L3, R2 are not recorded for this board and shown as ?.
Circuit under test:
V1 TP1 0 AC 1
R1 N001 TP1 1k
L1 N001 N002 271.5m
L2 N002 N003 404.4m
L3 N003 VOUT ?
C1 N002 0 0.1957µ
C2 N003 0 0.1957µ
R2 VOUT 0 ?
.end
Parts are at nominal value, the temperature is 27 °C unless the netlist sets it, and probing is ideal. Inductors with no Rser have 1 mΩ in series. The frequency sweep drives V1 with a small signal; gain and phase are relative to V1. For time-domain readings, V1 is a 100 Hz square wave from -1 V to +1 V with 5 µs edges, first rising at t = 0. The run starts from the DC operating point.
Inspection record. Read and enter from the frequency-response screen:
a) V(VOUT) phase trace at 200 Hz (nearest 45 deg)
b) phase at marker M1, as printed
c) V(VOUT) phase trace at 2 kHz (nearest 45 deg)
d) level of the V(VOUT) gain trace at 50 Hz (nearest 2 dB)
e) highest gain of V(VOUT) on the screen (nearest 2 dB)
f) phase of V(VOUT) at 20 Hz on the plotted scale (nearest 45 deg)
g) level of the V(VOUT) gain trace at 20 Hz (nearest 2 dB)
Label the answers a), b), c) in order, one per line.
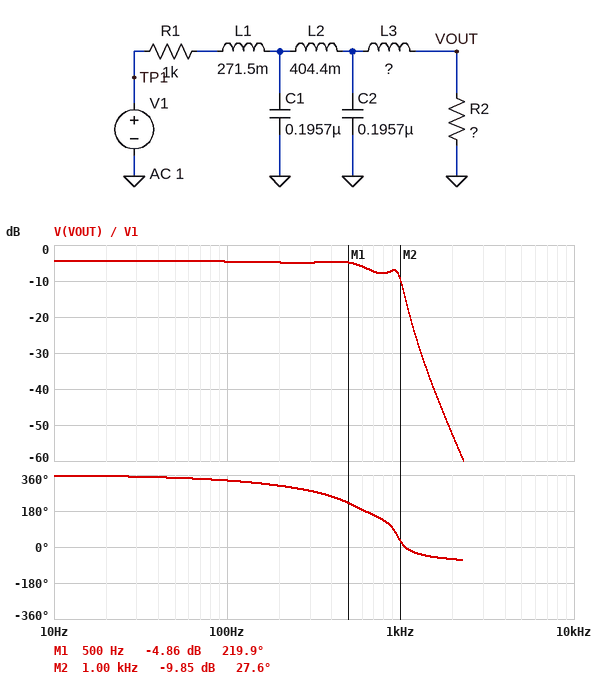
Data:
a) 315 deg
b) 219.9 deg
c) -45 deg
d) -4 dB
e) -4 dB
f) 360 deg
g) -4 dB
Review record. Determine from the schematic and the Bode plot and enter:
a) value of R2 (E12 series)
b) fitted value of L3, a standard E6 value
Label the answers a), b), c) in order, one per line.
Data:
a) 1.5 kΩ
b) 680 mH
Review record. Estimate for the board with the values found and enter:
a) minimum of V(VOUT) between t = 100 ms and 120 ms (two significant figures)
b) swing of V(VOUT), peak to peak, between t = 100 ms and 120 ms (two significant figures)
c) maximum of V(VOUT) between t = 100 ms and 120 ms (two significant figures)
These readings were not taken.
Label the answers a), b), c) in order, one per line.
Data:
a) -700 mV
b) 1.4 V
c) 700 mV
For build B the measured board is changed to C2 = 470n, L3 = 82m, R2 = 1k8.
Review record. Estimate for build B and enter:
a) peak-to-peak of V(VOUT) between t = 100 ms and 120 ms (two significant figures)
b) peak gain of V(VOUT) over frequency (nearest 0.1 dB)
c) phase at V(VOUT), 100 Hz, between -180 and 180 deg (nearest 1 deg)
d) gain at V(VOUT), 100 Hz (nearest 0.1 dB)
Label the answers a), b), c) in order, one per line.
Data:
a) 1.5 V
b) -3.6 dB
c) -26 deg
d) -3.7 dB
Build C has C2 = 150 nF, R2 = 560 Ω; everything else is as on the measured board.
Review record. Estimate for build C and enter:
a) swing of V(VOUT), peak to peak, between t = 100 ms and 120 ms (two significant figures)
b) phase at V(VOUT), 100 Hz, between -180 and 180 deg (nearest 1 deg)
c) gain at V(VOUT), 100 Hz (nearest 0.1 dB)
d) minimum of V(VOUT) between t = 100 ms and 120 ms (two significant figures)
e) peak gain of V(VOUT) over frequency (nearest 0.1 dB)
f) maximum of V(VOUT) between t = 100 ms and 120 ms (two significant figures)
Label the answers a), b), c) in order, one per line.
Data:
a) 740 mV
b) -34 deg
c) -9.6 dB
d) -370 mV
e) -8.9 dB
f) 370 mV
